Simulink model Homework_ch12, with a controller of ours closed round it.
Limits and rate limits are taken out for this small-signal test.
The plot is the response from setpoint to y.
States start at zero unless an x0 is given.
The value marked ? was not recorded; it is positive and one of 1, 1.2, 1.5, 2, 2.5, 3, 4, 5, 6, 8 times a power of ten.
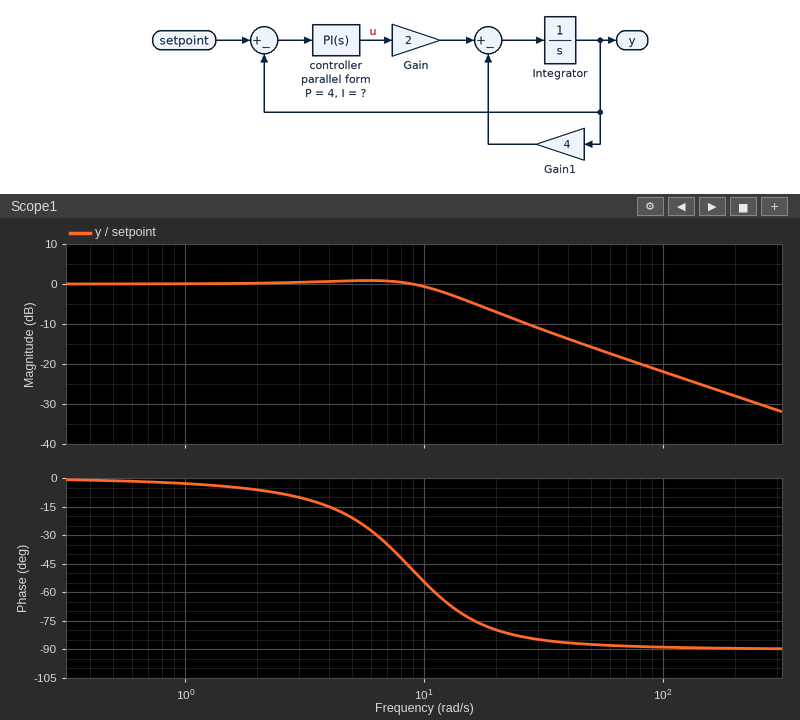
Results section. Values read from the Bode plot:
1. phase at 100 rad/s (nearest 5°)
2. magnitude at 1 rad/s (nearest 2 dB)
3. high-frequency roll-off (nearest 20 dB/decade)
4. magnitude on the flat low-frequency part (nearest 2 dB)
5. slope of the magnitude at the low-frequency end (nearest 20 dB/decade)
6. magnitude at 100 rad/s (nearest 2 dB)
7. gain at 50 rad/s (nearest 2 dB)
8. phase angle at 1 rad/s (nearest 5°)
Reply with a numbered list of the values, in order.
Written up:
1. -90°
2. 0 dB
3. -20 dB/decade
4. 0 dB
5. 0 dB/decade
6. -22 dB
7. -16 dB
8. -5°
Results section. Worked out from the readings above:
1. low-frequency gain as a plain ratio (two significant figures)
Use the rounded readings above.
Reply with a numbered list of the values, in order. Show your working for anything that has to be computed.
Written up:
1. 10^(0 / 20) = 1.0
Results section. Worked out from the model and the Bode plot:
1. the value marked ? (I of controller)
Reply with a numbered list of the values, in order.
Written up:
1. 40
